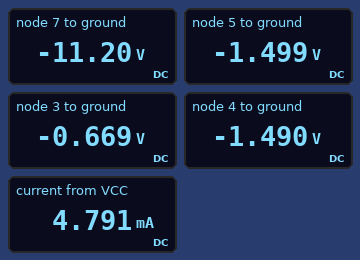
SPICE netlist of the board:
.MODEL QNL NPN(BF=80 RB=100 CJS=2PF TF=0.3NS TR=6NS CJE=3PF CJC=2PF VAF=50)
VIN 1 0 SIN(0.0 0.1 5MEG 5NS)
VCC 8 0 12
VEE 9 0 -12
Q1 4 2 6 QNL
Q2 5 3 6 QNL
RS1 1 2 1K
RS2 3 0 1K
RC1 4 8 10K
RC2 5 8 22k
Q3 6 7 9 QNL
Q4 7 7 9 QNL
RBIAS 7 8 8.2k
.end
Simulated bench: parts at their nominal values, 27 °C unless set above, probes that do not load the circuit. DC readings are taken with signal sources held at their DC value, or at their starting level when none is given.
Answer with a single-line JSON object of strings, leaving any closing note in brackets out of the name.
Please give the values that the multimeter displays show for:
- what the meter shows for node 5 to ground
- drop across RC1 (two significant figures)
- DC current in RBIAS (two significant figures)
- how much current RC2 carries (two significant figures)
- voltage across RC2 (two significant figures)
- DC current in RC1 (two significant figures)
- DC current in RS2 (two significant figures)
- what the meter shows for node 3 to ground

{"what the meter shows for node 5 to ground": "-1.499 V", "drop across RC1": "13 V", "DC current in RBIAS": "2.8 mA", "how much current RC2 carries": "610 µA", "voltage across RC2": "13 V", "DC current in RC1": "1.3 mA", "DC current in RS2": "670 µA", "what the meter shows for node 3 to ground": "-0.669 V"}
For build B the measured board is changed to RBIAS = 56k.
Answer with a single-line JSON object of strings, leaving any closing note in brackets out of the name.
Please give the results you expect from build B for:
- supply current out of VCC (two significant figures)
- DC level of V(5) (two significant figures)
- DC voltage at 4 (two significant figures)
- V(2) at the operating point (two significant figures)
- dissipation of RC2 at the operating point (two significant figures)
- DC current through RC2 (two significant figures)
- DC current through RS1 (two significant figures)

{"supply current out of VCC": "900 µA", "DC level of V(5)": "6.8 V", "DC voltage at 4": "9.5 V", "V(2) at the operating point": "-2.6 mV", "dissipation of RC2 at the operating point": "1.2 mW", "DC current through RC2": "240 µA", "DC current through RS1": "2.6 µA"}
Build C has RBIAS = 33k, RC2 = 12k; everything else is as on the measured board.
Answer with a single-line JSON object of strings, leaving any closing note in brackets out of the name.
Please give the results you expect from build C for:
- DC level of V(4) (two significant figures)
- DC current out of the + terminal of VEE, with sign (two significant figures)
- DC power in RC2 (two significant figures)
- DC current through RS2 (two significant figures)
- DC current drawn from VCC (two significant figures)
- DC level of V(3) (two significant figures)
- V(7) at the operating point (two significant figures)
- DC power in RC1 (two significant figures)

{"DC level of V(4)": "7.9 V", "DC current out of the + terminal of VEE, with sign": "-1.5 mA", "DC power in RC2": "2.0 mW", "DC current through RS2": "4.5 µA", "DC current drawn from VCC": "1.5 mA", "DC level of V(3)": "-4.5 mV", "V(7) at the operating point": "-11 V", "DC power in RC1": "1.7 mW"}
